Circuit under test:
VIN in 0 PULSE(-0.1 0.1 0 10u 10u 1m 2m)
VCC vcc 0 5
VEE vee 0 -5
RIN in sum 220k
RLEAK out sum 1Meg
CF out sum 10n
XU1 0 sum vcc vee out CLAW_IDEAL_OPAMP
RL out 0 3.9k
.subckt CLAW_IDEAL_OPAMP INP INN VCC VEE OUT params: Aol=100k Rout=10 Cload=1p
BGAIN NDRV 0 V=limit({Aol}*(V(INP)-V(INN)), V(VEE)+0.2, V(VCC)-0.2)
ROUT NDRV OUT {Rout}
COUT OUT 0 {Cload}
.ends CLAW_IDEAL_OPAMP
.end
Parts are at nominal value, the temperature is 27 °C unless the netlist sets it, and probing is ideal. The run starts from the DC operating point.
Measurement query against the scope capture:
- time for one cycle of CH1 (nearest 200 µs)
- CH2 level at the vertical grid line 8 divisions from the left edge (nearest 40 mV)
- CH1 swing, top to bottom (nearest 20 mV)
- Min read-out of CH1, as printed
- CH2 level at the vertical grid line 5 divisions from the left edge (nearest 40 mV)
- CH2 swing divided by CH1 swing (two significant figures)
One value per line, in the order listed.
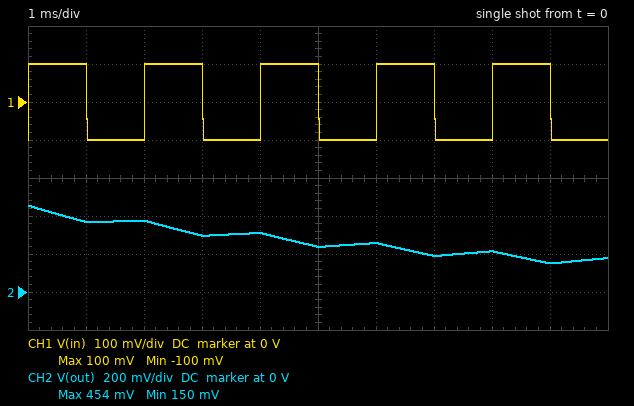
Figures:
2.0 ms
200 mV
200 mV
-100 mV
240 mV
1.5
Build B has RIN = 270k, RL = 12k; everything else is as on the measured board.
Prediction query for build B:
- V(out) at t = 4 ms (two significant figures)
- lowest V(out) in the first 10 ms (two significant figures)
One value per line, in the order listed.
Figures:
250 mV
120 mV
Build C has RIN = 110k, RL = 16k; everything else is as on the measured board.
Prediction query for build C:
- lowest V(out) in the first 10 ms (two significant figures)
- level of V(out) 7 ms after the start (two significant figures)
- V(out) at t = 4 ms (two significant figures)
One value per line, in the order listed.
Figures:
300 mV
380 mV
620 mV
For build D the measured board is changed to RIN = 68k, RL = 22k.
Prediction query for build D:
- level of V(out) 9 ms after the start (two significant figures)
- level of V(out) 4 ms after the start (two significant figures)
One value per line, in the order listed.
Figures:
490 mV
1.0 V
